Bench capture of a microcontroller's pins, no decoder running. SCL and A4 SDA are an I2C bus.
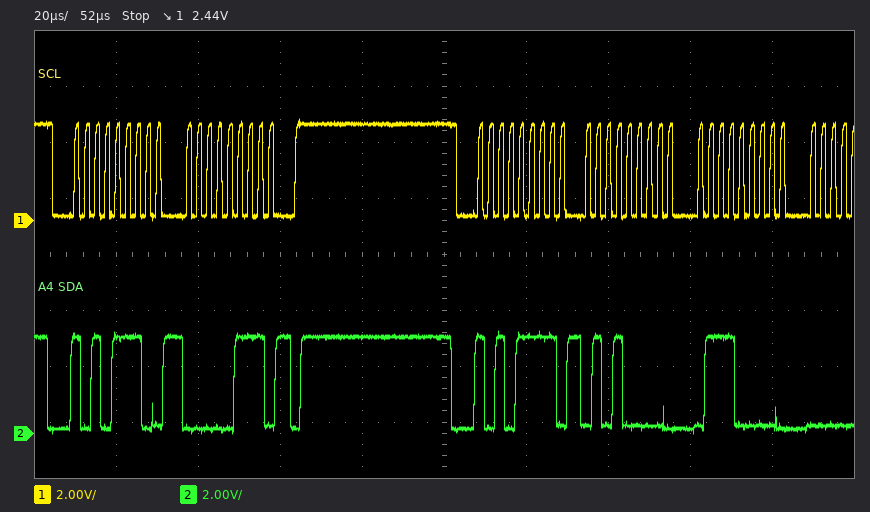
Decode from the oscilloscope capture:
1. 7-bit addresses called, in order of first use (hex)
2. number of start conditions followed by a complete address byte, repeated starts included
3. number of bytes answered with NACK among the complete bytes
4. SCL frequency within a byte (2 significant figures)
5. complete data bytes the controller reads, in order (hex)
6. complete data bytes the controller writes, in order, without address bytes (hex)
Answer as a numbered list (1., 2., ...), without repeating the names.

1. 0x57
2. 2
3. 0
4. 400 kHz
5. 50 70
6. 07
